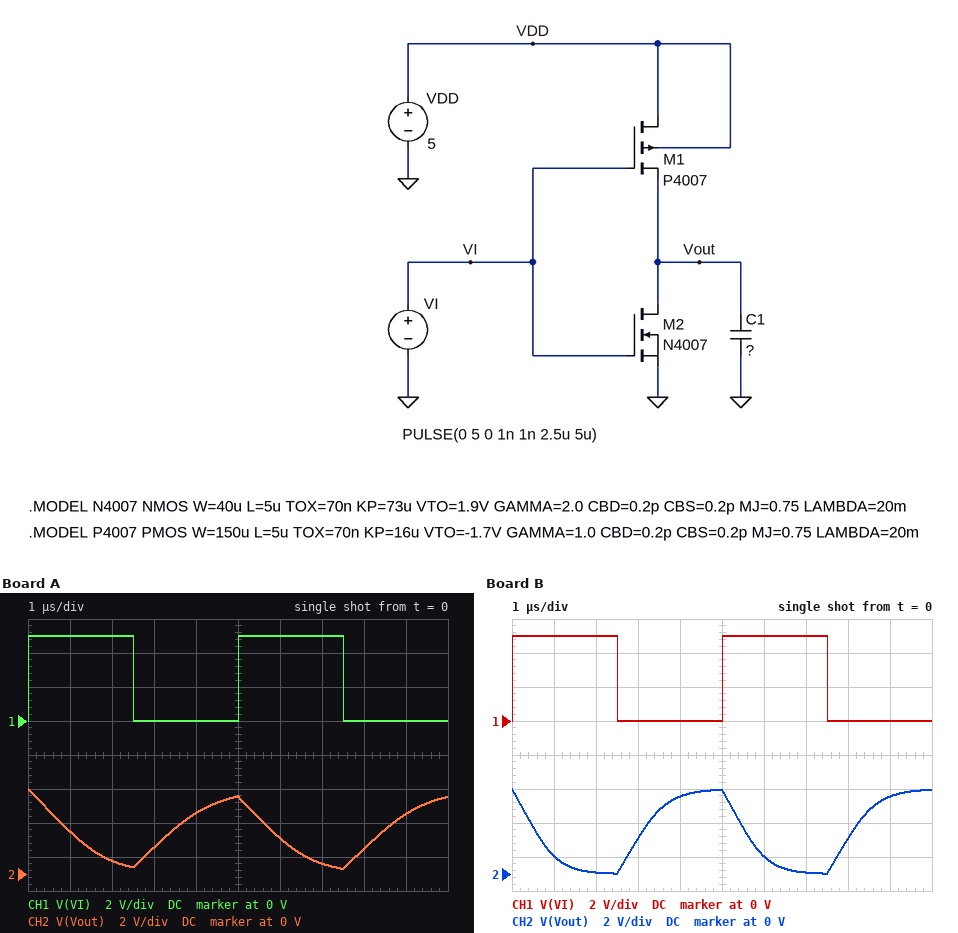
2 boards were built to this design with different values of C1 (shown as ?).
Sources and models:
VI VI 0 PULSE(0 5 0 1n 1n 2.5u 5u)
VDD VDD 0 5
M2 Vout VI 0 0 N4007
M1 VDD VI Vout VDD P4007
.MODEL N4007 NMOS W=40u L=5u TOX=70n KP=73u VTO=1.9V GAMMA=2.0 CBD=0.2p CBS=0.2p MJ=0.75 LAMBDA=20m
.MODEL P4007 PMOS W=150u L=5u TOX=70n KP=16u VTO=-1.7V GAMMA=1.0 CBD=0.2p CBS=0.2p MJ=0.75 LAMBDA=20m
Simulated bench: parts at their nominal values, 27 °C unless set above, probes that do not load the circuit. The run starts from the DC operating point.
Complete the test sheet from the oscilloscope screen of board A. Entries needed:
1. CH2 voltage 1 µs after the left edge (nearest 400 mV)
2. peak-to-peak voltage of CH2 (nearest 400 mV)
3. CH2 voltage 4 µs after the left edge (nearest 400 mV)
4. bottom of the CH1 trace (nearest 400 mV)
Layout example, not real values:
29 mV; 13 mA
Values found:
2.4 V; 4.8 V; 3.6 V; 0 V
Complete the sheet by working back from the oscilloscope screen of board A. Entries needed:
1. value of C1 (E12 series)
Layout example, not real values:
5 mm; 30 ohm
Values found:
1.2 nF
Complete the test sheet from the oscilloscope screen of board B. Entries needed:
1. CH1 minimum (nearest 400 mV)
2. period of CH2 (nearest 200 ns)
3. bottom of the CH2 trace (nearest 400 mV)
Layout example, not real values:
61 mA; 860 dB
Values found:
0 V; 5.0 µs; 0 V
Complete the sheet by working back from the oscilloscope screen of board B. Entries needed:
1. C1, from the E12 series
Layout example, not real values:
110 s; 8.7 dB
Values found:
680 pF
